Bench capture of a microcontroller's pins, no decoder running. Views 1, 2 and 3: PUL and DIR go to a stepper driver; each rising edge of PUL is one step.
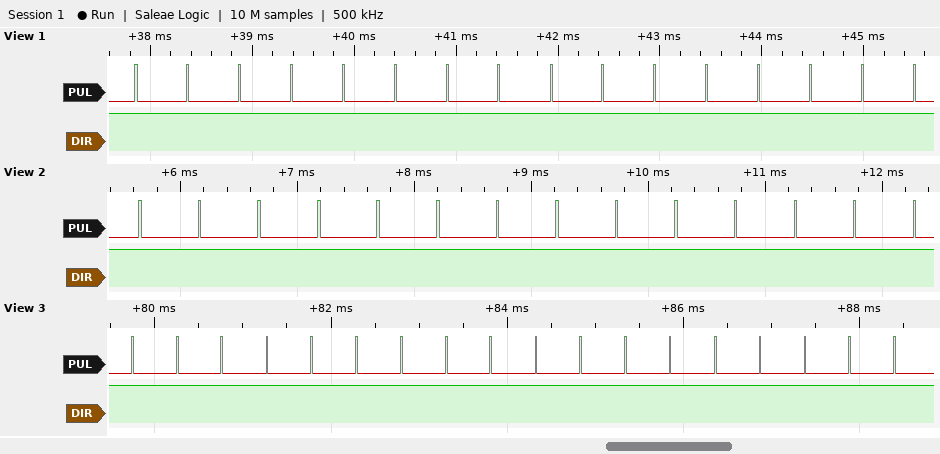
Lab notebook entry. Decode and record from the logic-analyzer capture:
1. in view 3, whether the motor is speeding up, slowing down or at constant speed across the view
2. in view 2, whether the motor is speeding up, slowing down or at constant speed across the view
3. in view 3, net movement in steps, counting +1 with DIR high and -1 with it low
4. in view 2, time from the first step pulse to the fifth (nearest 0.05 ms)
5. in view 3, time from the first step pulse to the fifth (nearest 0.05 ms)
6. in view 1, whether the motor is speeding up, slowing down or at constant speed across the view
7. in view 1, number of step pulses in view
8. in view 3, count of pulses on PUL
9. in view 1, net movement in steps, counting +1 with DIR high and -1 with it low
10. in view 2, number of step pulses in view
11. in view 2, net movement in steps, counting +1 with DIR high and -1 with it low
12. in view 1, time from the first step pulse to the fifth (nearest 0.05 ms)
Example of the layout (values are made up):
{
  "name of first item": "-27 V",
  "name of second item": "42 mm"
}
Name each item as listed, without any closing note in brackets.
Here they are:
{
  "in view 3, whether the motor is speeding up, slowing down or at constant speed across the view": "constant speed",
  "in view 2, whether the motor is speeding up, slowing down or at constant speed across the view": "constant speed",
  "in view 3, net movement in steps, counting +1 with DIR high and -1 with it low": "+18",
  "in view 2, time from the first step pulse to the fifth": "2.05 ms",
  "in view 3, time from the first step pulse to the fifth": "2.05 ms",
  "in view 1, whether the motor is speeding up, slowing down or at constant speed across the view": "constant speed",
  "in view 1, number of step pulses in view": "16",
  "in view 3, count of pulses on PUL": "18",
  "in view 1, net movement in steps, counting +1 with DIR high and -1 with it low": "+16",
  "in view 2, number of step pulses in view": "14",
  "in view 2, net movement in steps, counting +1 with DIR high and -1 with it low": "+14",
  "in view 1, time from the first step pulse to the fifth": "2.05 ms"
}
